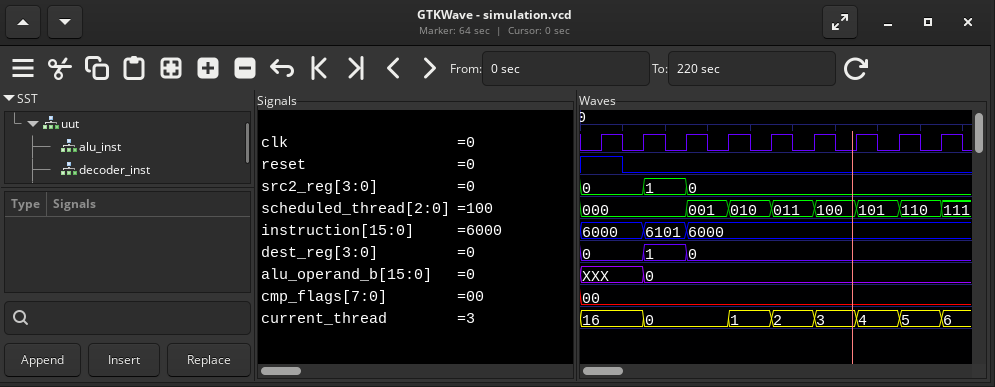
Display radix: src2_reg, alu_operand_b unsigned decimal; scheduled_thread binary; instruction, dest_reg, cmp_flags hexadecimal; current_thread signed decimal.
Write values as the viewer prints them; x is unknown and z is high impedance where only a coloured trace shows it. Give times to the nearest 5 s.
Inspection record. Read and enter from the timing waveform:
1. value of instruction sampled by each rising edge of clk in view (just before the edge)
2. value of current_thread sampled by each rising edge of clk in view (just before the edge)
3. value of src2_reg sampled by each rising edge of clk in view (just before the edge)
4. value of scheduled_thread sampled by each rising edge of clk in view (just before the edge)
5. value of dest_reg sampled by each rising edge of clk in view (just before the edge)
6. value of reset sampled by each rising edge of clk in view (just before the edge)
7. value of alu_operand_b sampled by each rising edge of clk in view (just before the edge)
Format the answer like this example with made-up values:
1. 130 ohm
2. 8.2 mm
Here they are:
1. 6000, 6000, 6101, 6000, 6000, 6000, 6000, 6000, 6000
2. 16, 16, 0, 0, 1, 2, 3, 4, 5
3. 0, 0, 1, 0, 0, 0, 0, 0, 0
4. 000, 000, 000, 001, 010, 011, 100, 101, 110
5. 0, 0, 1, 0, 0, 0, 0, 0, 0
6. 1 0 0 0 0 0 0 0 0
7. XXX, XXX, 0, 0, 0, 0, 0, 0, 0
